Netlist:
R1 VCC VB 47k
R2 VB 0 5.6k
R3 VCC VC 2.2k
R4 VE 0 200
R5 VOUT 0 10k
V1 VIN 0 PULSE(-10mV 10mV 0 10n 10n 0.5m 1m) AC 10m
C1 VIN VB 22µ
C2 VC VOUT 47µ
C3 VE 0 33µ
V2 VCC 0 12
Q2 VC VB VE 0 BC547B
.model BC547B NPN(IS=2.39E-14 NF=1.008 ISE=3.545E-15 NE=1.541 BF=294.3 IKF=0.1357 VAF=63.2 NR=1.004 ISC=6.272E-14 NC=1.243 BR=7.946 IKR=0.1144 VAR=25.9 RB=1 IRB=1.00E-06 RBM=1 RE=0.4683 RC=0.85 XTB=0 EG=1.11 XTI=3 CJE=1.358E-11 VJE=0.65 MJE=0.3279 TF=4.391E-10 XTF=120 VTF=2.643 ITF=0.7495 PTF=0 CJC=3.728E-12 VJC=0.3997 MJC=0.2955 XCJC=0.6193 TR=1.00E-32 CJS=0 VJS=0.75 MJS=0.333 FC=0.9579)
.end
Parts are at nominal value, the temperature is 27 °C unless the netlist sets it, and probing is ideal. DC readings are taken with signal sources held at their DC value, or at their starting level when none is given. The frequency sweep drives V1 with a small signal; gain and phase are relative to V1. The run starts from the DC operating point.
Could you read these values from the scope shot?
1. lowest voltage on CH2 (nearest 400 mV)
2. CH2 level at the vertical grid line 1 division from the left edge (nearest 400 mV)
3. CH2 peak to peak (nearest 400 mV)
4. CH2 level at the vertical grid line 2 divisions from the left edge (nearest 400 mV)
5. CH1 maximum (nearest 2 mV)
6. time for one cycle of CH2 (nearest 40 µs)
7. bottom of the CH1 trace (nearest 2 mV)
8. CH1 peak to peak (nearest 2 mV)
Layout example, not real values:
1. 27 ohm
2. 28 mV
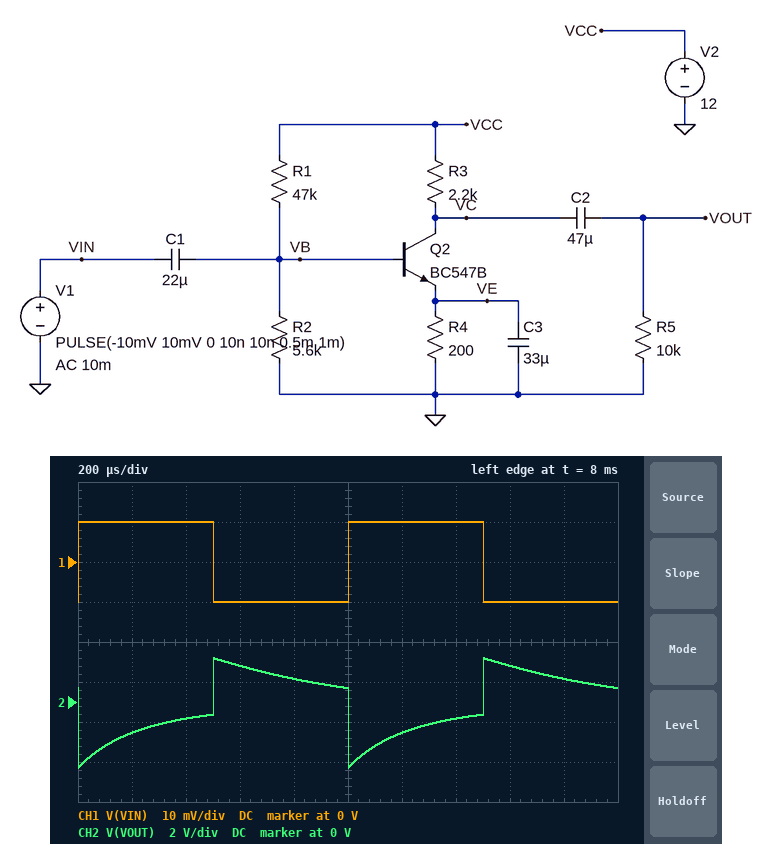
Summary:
1. -3.2 V
2. -1.6 V
3. 5.6 V
4. -800 mV
5. 10 mV
6. 1.00 ms
7. -10 mV
8. 20 mV
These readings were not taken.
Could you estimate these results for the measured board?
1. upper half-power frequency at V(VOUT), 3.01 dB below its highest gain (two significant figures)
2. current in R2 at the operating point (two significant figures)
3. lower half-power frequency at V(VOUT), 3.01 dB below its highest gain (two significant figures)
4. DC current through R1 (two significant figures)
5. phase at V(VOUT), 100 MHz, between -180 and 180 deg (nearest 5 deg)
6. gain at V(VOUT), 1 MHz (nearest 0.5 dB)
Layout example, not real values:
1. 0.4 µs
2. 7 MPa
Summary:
1. 50 MHz
2. 220 µA
3. 480 Hz
4. 230 µA
5. 110 deg
6. 44.5 dB
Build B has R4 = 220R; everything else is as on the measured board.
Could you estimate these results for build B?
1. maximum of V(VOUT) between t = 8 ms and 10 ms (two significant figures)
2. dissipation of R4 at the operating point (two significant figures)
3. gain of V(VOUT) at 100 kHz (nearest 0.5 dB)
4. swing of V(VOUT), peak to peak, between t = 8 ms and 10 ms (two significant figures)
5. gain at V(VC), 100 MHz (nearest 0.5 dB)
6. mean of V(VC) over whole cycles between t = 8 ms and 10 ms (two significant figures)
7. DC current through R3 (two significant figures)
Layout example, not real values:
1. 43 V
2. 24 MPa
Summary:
1. 2.0 V
2. 1.5 mW
3. 44.0 dB
4. 5.0 V
5. 37.0 dB
6. 6.2 V
7. 2.6 mA
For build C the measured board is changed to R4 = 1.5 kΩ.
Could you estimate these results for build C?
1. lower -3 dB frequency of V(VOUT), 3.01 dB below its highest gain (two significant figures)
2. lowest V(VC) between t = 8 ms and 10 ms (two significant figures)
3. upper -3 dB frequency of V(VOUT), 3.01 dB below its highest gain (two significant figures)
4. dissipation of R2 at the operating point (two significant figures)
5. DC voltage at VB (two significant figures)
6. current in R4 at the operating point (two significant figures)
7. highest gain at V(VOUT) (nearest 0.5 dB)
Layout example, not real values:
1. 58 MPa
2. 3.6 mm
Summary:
1. 83 Hz
2. 11 V
3. 62 MHz
4. 290 µW
5. 1.3 V
6. 440 µA
7. 29.5 dB
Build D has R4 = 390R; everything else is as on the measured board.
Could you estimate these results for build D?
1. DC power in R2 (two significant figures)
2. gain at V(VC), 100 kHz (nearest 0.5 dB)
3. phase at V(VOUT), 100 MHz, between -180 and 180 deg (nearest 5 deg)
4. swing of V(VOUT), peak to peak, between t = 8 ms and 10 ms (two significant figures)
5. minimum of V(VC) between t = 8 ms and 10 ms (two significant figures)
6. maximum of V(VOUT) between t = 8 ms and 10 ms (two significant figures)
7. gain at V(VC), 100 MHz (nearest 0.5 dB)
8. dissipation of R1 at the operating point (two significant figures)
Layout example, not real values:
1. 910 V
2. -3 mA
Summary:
1. 280 µW
2. 40.0 dB
3. 115 deg
4. 2.8 V
5. 7.0 V
6. 1.2 V
7. 34.0 dB
8. 2.5 mW
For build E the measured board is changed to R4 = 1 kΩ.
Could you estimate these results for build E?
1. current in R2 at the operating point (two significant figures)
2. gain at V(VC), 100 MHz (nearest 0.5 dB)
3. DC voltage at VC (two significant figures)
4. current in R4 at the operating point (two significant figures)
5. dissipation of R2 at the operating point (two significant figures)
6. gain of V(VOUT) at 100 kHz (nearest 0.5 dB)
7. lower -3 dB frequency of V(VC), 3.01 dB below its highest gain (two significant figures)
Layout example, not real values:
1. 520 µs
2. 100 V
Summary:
1. 230 µA
2. 27.0 dB
3. 11 V
4. 640 µA
5. 290 µW
6. 32.5 dB
7. 120 Hz
